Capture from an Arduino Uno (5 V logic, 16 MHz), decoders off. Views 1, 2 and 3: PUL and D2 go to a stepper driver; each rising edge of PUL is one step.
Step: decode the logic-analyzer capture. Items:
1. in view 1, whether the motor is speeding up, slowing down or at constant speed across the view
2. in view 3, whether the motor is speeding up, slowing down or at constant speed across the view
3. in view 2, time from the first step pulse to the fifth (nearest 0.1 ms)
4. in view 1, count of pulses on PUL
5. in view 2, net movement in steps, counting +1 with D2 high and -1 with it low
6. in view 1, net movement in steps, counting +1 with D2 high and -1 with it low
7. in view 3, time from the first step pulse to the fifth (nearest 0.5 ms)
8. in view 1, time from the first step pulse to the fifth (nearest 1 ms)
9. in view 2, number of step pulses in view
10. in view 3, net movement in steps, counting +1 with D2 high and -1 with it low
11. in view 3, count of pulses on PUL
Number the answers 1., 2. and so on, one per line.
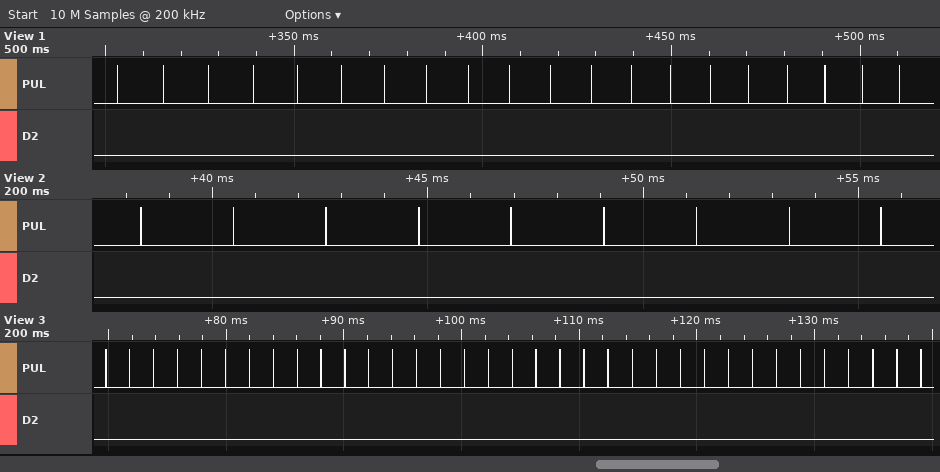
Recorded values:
1. speeding up
2. constant speed
3. 8.6 ms
4. 20
5. -9
6. -20
7. 8.0 ms
8. 48 ms
9. 9
10. -35
11. 35
